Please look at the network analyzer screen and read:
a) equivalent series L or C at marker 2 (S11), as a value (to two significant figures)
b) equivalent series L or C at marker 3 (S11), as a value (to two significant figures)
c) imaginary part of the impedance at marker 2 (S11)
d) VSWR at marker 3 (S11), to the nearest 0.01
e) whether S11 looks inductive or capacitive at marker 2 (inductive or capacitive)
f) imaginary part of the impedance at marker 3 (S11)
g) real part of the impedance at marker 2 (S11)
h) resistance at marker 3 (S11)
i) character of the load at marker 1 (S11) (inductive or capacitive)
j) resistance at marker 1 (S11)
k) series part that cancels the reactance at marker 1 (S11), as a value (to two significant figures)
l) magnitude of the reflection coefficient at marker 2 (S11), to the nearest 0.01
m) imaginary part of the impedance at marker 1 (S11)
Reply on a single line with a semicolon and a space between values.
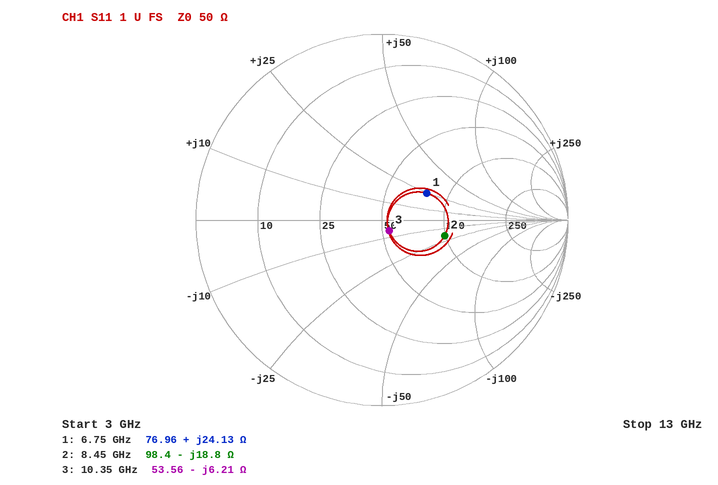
1.00 pF; 2.5 pF; -18.8 Ω; 1.15; capacitive; -6.21 Ω; 98.4 Ω; 53.56 Ω; inductive; 76.96 Ω; 980 fF; 0.35; +24.13 Ω
